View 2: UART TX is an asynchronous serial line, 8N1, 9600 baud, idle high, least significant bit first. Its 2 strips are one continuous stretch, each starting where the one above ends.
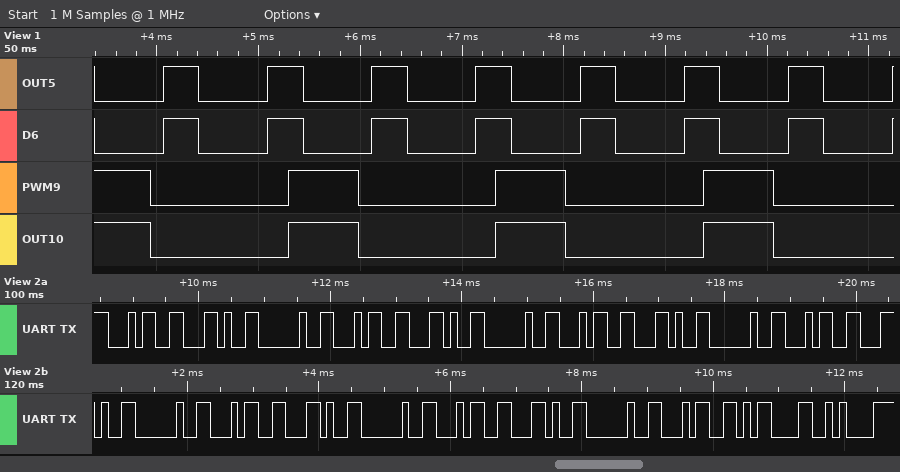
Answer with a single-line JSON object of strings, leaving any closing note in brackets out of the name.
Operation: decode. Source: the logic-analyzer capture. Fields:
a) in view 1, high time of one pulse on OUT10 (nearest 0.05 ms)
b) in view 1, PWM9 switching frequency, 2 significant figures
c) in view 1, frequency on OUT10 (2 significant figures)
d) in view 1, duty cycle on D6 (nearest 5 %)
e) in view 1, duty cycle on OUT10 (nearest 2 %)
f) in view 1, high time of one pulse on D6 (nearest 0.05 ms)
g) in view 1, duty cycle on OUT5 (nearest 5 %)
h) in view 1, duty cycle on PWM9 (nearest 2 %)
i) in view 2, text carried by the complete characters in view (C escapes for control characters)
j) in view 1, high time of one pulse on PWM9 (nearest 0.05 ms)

{"in view 1, high time of one pulse on OUT10": "0.70 ms", "in view 1, PWM9 switching frequency, 2 significant figures": "490 Hz", "in view 1, frequency on OUT10": "490 Hz", "in view 1, duty cycle on D6": "35 %", "in view 1, duty cycle on OUT10": "34 %", "in view 1, high time of one pulse on D6": "0.35 ms", "in view 1, duty cycle on OUT5": "35 %", "in view 1, duty cycle on PWM9": "34 %", "in view 2, text carried by the complete characters in view": "\"4, 4, 4, 4, 4, 4, 4\\r\\n\"", "in view 1, high time of one pulse on PWM9": "0.70 ms"}
